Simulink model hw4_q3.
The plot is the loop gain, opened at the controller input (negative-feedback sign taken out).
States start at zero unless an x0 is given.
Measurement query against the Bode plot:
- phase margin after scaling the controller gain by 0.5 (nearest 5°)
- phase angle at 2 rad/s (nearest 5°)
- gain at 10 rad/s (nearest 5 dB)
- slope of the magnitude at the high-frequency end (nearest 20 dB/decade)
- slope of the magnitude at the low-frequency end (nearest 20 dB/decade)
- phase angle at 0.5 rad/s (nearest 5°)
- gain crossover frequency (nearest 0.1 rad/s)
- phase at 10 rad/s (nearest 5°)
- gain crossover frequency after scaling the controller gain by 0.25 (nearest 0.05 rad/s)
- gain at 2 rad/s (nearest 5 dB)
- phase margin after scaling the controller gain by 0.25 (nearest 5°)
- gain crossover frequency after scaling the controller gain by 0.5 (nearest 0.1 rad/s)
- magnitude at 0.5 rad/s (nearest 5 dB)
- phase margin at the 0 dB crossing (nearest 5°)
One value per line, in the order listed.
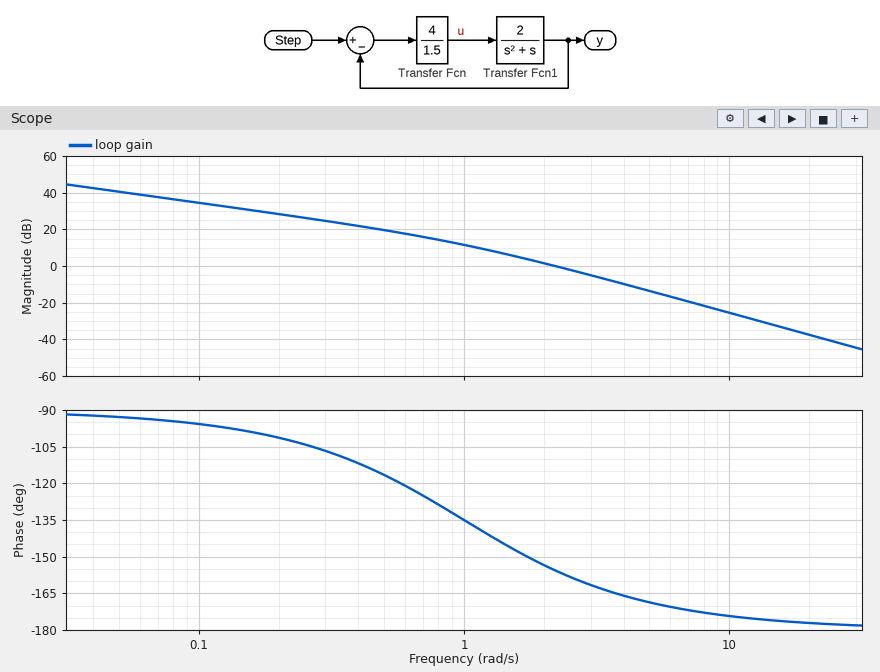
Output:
35°
-155°
-25 dB
-40 dB/decade
-20 dB/decade
-115°
2.2 rad/s
-175°
0.95 rad/s
0 dB
45°
1.5 rad/s
20 dB
25°
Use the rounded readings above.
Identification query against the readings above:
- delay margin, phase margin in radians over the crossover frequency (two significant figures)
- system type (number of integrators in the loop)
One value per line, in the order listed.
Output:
0.20 s
1
